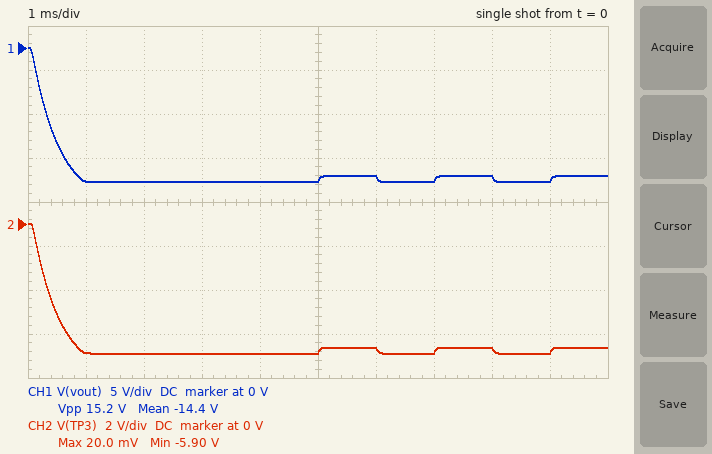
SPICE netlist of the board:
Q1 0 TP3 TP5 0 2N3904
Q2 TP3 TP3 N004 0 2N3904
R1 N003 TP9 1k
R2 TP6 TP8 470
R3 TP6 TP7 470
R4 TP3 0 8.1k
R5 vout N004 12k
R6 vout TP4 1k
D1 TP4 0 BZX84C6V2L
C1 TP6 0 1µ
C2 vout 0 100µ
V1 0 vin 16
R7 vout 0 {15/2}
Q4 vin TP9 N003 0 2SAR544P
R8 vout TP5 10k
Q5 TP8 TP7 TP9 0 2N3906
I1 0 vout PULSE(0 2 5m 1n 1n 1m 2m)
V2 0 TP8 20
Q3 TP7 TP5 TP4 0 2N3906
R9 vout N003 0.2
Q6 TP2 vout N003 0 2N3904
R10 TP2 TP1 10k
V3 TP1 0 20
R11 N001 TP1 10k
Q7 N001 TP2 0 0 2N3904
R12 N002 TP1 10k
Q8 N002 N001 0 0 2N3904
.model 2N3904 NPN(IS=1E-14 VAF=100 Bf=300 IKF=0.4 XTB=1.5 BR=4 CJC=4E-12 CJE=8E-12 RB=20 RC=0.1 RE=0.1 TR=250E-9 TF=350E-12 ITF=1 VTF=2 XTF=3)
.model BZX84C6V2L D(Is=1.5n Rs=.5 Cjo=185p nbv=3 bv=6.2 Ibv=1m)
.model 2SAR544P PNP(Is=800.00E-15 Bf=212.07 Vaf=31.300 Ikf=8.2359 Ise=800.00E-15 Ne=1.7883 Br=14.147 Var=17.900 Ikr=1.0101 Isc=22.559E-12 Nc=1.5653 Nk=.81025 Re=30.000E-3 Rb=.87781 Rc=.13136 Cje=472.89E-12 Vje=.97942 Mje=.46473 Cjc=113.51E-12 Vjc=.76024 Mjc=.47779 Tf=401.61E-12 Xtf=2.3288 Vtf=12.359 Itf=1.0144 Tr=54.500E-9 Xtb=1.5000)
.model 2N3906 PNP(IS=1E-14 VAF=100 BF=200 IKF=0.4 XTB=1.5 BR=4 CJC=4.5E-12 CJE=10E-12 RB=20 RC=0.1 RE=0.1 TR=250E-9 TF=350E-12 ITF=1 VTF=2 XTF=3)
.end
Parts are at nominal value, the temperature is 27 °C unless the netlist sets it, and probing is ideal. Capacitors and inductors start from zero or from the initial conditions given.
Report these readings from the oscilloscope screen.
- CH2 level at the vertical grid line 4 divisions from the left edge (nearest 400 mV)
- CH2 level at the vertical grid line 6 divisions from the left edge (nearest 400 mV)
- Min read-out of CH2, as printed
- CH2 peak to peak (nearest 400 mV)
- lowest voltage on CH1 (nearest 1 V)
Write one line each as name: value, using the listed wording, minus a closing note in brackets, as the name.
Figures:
CH2 level at the vertical grid line 4 divisions from the left edge: -6.0 V
CH2 level at the vertical grid line 6 divisions from the left edge: -5.6 V
Min read-out of CH2, as printed: -5.90 V
CH2 peak to peak: 6.0 V
lowest voltage on CH1: -15 V
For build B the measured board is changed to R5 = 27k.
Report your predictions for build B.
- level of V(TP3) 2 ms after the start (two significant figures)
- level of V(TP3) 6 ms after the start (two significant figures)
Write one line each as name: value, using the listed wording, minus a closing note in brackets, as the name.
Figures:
level of V(TP3) 2 ms after the start: -3.4 V
level of V(TP3) 6 ms after the start: -3.2 V
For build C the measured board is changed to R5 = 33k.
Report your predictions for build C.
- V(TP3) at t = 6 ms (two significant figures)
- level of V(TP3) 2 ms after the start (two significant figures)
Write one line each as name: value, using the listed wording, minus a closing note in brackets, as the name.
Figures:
V(TP3) at t = 6 ms: -2.8 V
level of V(TP3) 2 ms after the start: -2.9 V
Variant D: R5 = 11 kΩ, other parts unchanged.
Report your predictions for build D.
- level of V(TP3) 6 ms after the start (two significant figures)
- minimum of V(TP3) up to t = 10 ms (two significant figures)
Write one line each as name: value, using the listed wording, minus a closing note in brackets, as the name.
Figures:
level of V(TP3) 6 ms after the start: -5.9 V
minimum of V(TP3) up to t = 10 ms: -6.2 V
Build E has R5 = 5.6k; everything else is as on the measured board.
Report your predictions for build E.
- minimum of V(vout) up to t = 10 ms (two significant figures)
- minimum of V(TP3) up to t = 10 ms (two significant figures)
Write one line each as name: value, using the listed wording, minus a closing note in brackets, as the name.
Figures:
minimum of V(vout) up to t = 10 ms: -12 V
minimum of V(TP3) up to t = 10 ms: -6.5 V
